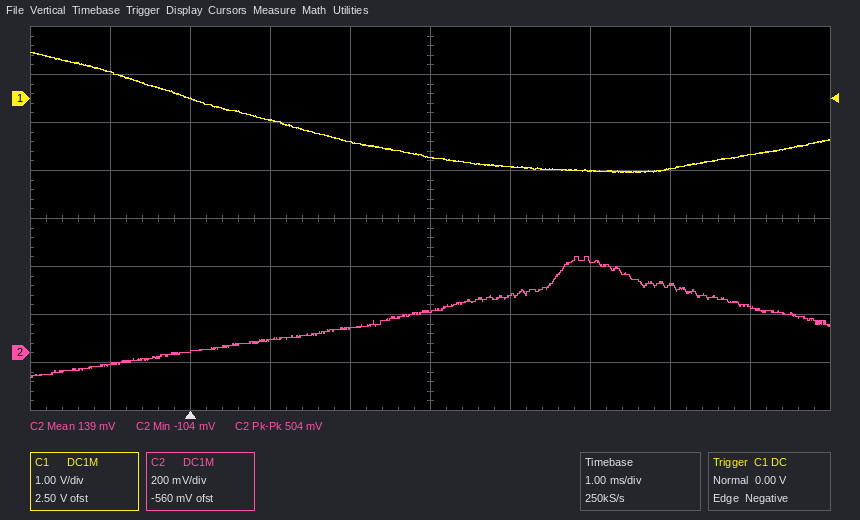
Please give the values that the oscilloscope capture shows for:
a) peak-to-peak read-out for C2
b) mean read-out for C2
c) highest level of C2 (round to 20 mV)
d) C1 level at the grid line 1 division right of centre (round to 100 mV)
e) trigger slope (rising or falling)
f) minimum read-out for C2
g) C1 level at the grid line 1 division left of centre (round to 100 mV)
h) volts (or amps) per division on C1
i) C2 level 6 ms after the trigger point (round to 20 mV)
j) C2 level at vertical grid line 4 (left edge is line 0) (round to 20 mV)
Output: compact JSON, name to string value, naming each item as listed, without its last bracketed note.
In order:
{"peak-to-peak read-out for C2": "504 mV", "mean read-out for C2": "139 mV", "highest level of C2": "400 mV", "C1 level at the grid line 1 division right of centre": "-1.4 V", "trigger slope": "falling", "minimum read-out for C2": "-104 mV", "C1 level at the grid line 1 division left of centre": "-900 mV", "volts (or amps) per division on C1": "1 V", "C2 level 6 ms after the trigger point": "280 mV", "C2 level at vertical grid line 4 (left edge is line 0)": "100 mV"}
